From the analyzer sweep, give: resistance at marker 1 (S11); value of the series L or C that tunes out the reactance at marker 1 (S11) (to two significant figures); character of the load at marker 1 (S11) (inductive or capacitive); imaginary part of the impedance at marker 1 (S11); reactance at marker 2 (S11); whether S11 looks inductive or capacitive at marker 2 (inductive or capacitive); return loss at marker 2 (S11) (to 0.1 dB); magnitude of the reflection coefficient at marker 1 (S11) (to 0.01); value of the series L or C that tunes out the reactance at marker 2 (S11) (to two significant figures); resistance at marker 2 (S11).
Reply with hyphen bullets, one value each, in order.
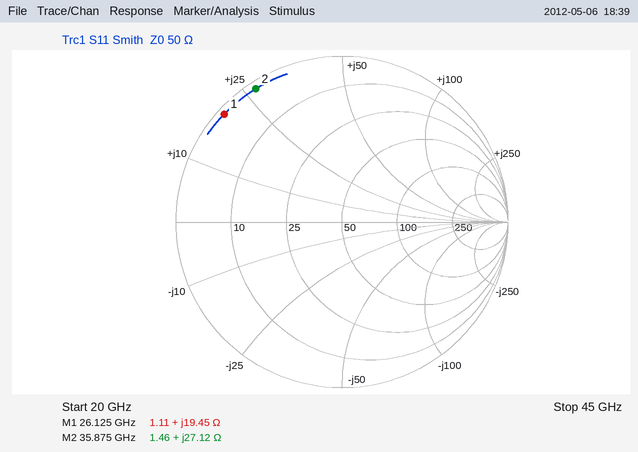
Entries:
- 1.11 Ω
- 310 fF
- inductive
- +19.45 Ω
- +27.12 Ω
- inductive
- 0.4 dB
- 0.96
- 160 fF
- 1.46 Ω
